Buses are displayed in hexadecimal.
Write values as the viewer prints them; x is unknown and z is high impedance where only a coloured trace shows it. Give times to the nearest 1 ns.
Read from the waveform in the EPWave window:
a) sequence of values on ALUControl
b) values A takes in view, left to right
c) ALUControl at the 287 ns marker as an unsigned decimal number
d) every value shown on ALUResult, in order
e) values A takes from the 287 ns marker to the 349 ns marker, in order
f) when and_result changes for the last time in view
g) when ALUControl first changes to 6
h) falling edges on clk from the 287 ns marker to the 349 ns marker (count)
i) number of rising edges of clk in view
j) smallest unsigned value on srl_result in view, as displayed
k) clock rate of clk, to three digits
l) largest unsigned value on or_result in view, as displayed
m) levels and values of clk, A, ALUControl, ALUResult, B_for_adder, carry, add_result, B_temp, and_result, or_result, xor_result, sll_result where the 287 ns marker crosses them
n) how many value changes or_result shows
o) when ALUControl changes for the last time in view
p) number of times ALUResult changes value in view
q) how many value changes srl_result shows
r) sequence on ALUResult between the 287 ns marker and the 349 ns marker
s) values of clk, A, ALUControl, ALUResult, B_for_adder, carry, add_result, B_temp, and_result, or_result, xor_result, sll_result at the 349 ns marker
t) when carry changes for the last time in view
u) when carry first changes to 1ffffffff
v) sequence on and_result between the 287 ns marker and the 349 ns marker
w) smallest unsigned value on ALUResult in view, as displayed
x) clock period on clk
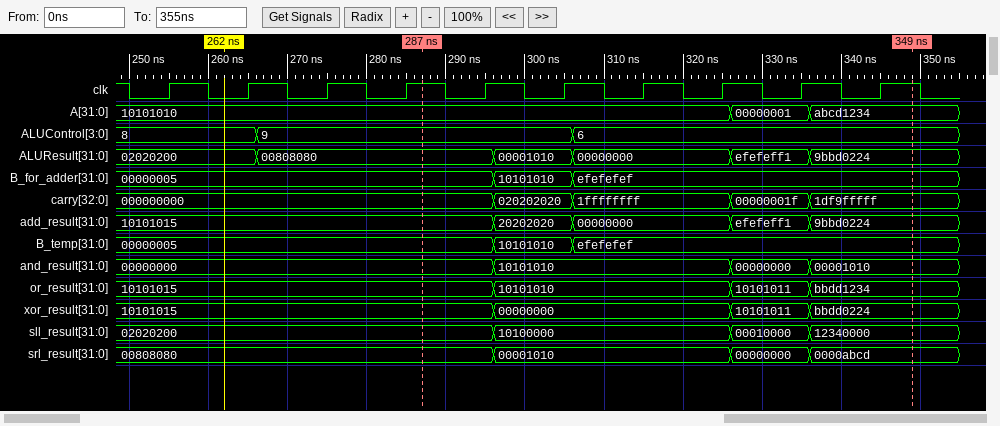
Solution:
8, 9, 6
10101010, 00000001, abcd1234
9
02020200, 00808080, 00001010, 00000000, efefeff1, 9bbd0224
10101010, 00000001, abcd1234
336 ns
306 ns
6
10
00000000
100 MHz
bbdd1234
clk=1, A=10101010, ALUControl=9, ALUResult=00808080, B_for_adder=00000005, carry=000000000, add_result=10101015, B_temp=00000005, and_result=00000000, or_result=10101015, xor_result=10101015, sll_result=02020200
3
306 ns
5
3
00808080, 00001010, 00000000, efefeff1, 9bbd0224
clk=1, A=abcd1234, ALUControl=6, ALUResult=9bbd0224, B_for_adder=efefefef, carry=1df9fffff, add_result=9bbd0224, B_temp=efefefef, and_result=00001010, or_result=bbdd1234, xor_result=bbdd0224, sll_result=12340000
336 ns
306 ns
00000000, 10101010, 00000000, 00001010
00000000
10 ns
